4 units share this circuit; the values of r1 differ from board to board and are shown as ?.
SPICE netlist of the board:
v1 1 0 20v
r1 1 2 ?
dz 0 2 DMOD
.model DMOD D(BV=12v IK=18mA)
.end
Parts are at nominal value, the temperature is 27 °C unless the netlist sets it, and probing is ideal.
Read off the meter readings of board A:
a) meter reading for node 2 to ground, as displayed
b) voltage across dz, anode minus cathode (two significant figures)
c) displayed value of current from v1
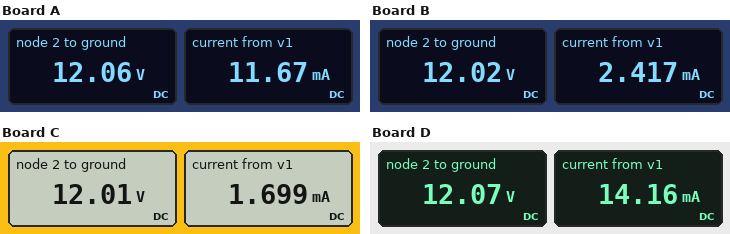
12.06 V
-12 V
11.67 mA
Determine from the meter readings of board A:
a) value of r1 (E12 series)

680 Ω
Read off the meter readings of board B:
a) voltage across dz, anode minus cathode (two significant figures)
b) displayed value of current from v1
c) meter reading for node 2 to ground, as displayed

-12 V
2.417 mA
12.02 V
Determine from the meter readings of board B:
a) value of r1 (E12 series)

3.3 kΩ
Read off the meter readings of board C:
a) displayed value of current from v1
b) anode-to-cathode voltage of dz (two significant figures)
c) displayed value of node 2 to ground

1.699 mA
-12 V
12.01 V
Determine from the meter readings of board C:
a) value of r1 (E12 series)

4.7 kΩ
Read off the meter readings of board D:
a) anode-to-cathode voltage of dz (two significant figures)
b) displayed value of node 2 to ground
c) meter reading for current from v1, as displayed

-12 V
12.07 V
14.16 mA
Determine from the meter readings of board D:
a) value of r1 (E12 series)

560 Ω
